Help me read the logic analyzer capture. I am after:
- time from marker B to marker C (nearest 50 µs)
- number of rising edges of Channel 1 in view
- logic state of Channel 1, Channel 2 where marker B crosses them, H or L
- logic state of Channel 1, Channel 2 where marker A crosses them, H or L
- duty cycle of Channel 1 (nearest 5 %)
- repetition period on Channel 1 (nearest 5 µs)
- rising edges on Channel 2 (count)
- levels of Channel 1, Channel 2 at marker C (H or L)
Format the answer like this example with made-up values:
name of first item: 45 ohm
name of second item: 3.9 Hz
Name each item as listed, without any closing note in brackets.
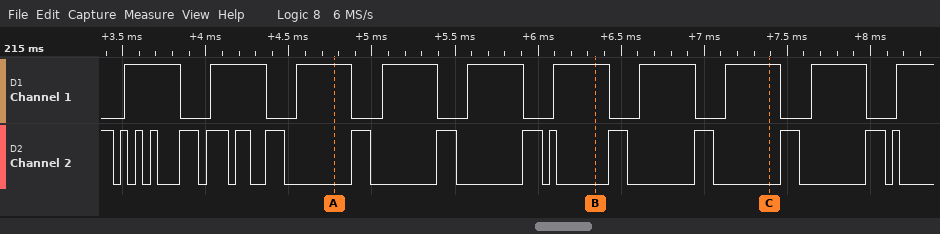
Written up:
time from marker B to marker C: 1050 µs
number of rising edges of Channel 1 in view: 10
logic state of Channel 1, Channel 2 where marker B crosses them, H or L: Channel 1=H, Channel 2=L
logic state of Channel 1, Channel 2 where marker A crosses them, H or L: Channel 1=H, Channel 2=L
duty cycle of Channel 1: 65 %
repetition period on Channel 1: 515 µs
rising edges on Channel 2: 16
levels of Channel 1, Channel 2 at marker C: Channel 1=H, Channel 2=L
